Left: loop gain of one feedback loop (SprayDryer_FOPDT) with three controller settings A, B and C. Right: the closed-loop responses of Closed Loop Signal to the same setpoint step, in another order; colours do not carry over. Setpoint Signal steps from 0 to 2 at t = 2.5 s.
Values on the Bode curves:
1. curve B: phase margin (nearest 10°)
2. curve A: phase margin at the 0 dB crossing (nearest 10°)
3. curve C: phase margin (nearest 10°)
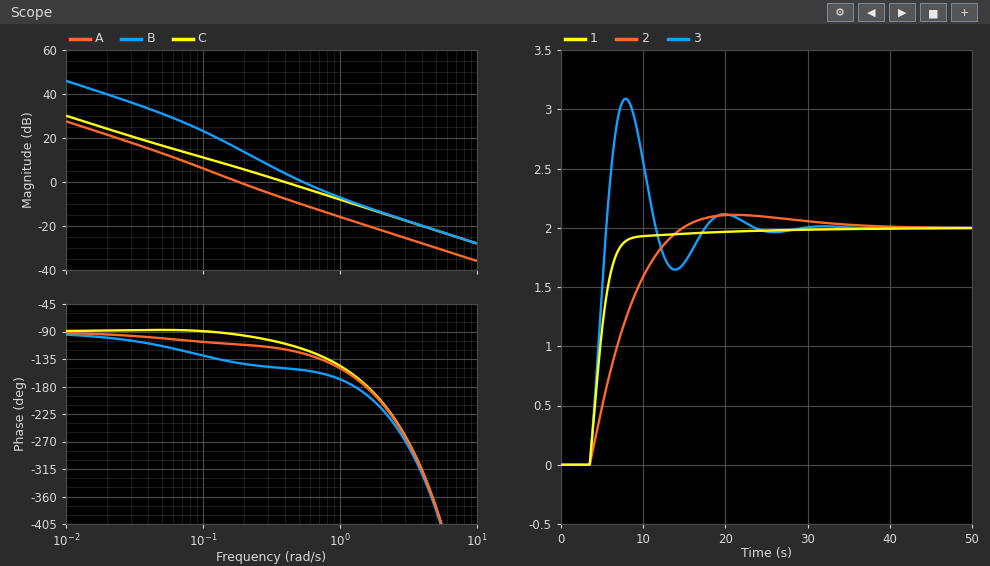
30°
70°
70°
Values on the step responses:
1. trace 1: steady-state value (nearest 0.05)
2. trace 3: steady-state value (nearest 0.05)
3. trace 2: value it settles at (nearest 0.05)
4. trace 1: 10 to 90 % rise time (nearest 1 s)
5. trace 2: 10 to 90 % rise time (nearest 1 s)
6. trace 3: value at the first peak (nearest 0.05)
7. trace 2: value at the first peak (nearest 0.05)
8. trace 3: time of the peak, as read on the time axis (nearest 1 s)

2.00
2.00
2.00
3 s
8 s
3.10
2.10
8 s
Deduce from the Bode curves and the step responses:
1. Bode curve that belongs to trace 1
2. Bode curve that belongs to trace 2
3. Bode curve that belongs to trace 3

C
A
B
